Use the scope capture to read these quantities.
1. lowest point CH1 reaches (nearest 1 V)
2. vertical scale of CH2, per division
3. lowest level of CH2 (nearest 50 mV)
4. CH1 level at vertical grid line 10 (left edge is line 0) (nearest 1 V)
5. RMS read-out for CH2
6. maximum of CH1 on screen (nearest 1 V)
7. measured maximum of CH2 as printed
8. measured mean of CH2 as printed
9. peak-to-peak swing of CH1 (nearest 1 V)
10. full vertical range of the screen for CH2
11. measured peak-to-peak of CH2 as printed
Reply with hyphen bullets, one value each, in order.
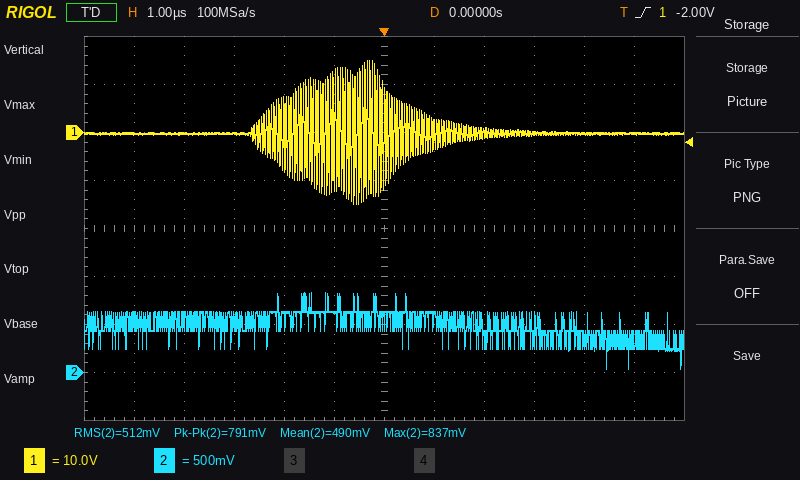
- -15 V
- 500 mV
- 50 mV
- 0 V
- 512 mV
- 15 V
- 837 mV
- 490 mV
- 30 V
- 4 V
- 791 mV
